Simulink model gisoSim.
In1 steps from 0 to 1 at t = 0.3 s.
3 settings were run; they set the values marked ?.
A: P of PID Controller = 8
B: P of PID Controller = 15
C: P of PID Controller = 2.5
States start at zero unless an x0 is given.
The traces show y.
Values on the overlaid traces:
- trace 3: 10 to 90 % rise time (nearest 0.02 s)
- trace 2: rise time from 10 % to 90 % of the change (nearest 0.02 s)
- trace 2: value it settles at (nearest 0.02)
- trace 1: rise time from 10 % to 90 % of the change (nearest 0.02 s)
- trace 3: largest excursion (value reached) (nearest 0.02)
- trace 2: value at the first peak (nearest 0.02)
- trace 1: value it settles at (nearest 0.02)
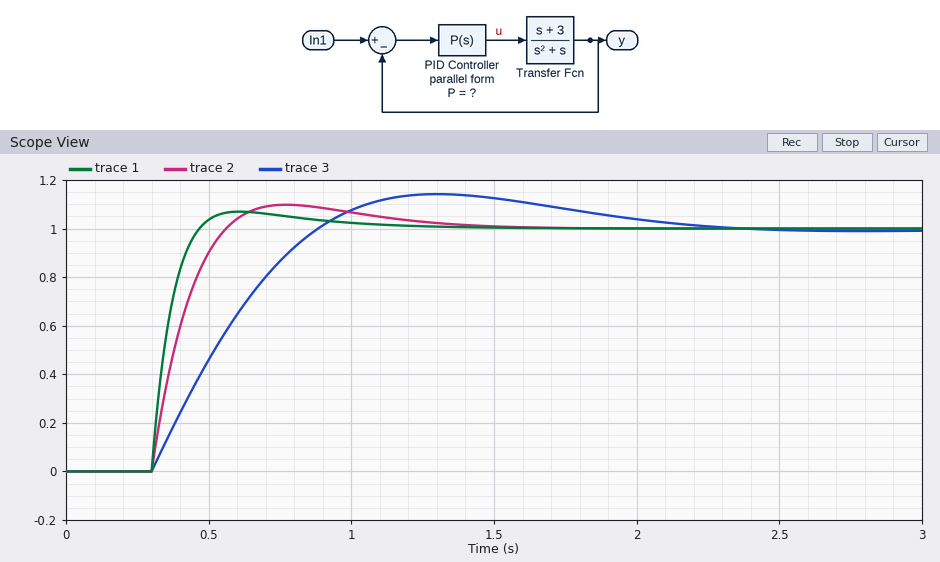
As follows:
0.44 s
0.18 s
1.00
0.12 s
1.14
1.10
1.00
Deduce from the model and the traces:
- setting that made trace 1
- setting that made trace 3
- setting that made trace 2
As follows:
B
C
A
